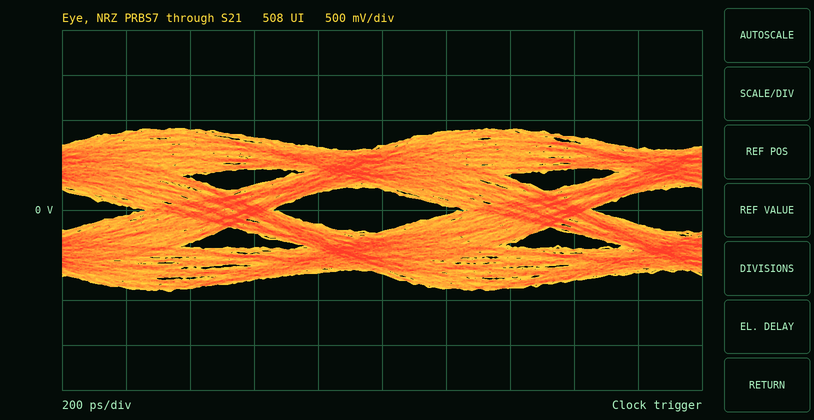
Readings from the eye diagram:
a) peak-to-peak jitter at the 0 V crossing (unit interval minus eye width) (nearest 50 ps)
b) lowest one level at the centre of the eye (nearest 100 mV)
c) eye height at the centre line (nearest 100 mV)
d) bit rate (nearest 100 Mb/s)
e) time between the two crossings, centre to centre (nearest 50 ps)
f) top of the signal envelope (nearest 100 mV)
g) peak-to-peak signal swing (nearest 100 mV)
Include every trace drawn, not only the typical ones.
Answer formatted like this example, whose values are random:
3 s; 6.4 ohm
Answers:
400 ps; 200 mV; 500 mV; 1.0 Gb/s; 1.00 ns; 900 mV; 1.8 V
